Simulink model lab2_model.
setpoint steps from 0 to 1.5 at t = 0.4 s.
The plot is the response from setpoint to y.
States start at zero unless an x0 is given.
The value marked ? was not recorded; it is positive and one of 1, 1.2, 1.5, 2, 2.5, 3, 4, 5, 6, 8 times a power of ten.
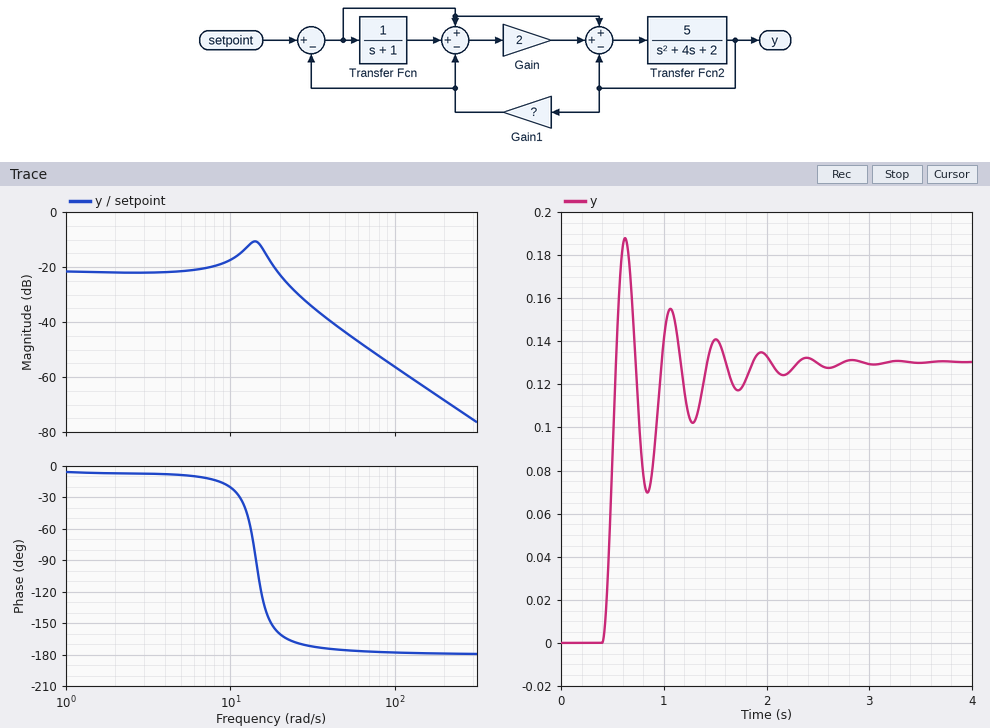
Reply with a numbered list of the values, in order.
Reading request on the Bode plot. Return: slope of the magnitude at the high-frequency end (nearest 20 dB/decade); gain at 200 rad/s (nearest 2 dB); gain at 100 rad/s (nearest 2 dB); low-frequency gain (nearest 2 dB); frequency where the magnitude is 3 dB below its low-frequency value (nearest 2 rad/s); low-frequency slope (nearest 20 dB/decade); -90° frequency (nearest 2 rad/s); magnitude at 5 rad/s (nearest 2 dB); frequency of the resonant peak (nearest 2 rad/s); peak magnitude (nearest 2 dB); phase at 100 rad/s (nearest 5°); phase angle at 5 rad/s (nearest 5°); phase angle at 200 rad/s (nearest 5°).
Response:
1. -40 dB/decade
2. -68 dB
3. -56 dB
4. -22 dB
5. 22 rad/s
6. 0 dB/decade
7. 14 rad/s
8. -22 dB
9. 14 rad/s
10. -10 dB
11. -180°
12. -10°
13. -180°
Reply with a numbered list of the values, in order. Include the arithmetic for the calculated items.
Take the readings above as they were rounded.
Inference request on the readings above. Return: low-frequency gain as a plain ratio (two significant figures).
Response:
1. 10^(-22 / 20) = 0.079
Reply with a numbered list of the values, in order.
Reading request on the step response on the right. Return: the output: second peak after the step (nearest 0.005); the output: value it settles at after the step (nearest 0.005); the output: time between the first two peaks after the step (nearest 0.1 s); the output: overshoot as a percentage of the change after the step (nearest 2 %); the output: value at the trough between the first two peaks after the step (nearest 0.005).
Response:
1. 0.155
2. 0.130
3. 0.4 s
4. 44 %
5. 0.070
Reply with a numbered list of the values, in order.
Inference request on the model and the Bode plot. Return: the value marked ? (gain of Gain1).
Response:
1. 8
